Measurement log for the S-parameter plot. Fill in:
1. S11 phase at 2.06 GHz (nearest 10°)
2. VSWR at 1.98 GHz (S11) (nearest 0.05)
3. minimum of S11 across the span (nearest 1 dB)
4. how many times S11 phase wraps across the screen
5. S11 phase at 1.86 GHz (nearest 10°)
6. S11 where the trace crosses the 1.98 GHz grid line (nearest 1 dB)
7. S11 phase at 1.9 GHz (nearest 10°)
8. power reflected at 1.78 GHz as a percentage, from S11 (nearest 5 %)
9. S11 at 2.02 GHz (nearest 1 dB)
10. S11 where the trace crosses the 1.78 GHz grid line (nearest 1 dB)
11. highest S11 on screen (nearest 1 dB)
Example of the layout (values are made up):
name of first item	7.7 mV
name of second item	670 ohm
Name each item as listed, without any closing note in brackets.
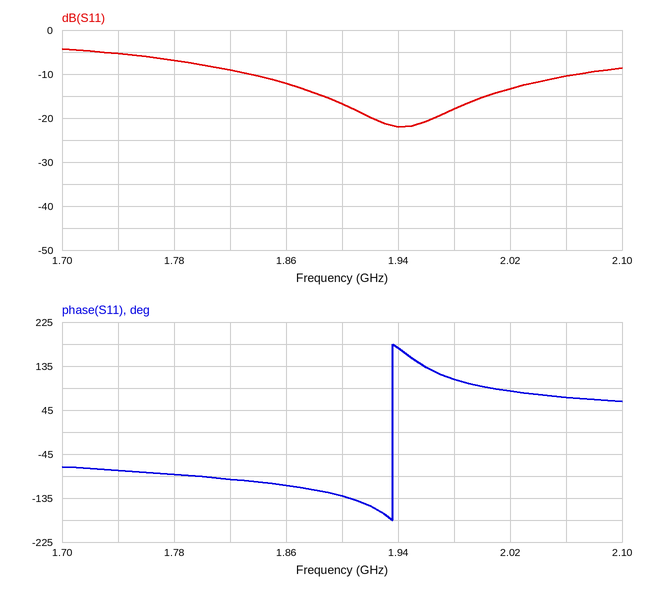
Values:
S11 phase at 2.06 GHz	70°
VSWR at 1.98 GHz (S11)	1.30
minimum of S11 across the span	-22 dB
how many times S11 phase wraps across the screen	1
S11 phase at 1.86 GHz	-110°
S11 where the trace crosses the 1.98 GHz grid line	-18 dB
S11 phase at 1.9 GHz	-130°
power reflected at 1.78 GHz as a percentage, from S11	20 %
S11 at 2.02 GHz	-13 dB
S11 where the trace crosses the 1.78 GHz grid line	-7 dB
highest S11 on screen	-4 dB
